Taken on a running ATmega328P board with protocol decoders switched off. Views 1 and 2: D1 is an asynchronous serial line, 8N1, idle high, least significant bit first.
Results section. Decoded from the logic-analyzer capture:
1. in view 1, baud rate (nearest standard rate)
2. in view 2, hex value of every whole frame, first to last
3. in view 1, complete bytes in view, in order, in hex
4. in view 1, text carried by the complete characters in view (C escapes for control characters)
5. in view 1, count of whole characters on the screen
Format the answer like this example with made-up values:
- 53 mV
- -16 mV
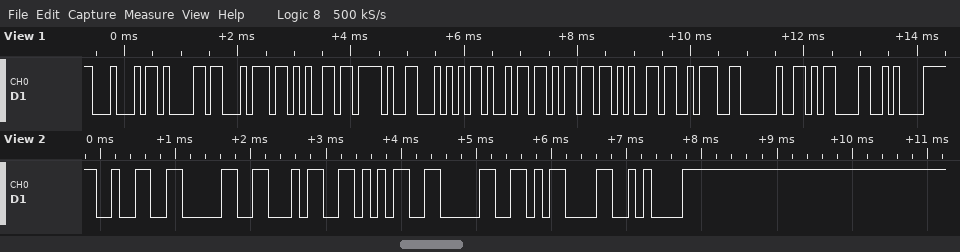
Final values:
- 9600 baud
- 32 30 34 35 30 0D 0A
- 44 61 74 65 2F 54 69 6D 65 3A 20 0D 0A
- "Date/Time: \r\n"
- 13
